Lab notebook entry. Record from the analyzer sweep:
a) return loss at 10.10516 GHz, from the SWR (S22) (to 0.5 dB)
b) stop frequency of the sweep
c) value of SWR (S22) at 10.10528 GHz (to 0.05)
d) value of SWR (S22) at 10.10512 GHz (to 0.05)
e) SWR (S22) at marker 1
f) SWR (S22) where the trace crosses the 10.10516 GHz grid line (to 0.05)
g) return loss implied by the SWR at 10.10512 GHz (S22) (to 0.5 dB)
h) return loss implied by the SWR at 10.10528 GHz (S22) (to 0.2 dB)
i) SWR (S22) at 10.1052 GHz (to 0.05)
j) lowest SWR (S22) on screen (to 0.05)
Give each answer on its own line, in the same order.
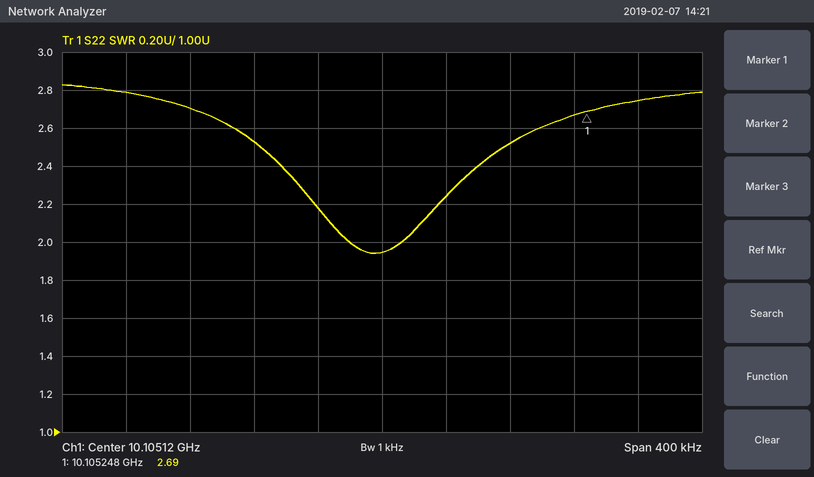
8.5 dB
10.10532 GHz
2.75
1.95
2.69
2.25
10.0 dB
6.6 dB
2.50
1.95
